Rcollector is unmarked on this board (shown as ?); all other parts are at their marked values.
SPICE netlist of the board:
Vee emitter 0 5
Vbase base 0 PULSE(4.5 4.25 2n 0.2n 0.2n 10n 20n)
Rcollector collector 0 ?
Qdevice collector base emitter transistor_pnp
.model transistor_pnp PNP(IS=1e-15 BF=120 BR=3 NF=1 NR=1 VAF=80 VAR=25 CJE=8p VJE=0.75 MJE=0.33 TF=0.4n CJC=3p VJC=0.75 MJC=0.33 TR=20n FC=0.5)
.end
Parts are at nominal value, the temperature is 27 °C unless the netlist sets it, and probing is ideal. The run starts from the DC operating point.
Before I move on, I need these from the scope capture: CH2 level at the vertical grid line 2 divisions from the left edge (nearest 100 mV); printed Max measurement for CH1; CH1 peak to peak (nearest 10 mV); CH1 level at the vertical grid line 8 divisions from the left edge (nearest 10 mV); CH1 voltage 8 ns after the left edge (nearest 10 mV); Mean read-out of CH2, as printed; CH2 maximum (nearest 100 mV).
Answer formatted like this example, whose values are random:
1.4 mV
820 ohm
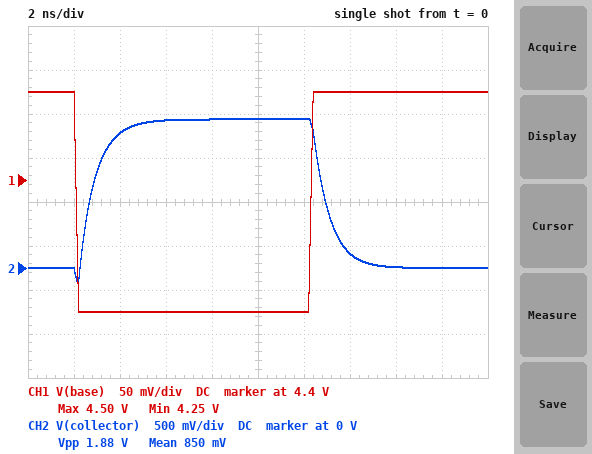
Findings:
1.5 V
4.50 V
250 mV
4.50 V
4.25 V
850 mV
1.7 V
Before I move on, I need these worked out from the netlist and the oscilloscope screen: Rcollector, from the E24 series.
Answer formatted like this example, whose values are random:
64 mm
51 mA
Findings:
430 Ω
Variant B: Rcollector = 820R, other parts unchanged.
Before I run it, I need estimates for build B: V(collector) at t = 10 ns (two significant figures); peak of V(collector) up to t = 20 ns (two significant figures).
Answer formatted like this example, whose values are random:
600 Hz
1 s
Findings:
3.1 V
3.2 V
